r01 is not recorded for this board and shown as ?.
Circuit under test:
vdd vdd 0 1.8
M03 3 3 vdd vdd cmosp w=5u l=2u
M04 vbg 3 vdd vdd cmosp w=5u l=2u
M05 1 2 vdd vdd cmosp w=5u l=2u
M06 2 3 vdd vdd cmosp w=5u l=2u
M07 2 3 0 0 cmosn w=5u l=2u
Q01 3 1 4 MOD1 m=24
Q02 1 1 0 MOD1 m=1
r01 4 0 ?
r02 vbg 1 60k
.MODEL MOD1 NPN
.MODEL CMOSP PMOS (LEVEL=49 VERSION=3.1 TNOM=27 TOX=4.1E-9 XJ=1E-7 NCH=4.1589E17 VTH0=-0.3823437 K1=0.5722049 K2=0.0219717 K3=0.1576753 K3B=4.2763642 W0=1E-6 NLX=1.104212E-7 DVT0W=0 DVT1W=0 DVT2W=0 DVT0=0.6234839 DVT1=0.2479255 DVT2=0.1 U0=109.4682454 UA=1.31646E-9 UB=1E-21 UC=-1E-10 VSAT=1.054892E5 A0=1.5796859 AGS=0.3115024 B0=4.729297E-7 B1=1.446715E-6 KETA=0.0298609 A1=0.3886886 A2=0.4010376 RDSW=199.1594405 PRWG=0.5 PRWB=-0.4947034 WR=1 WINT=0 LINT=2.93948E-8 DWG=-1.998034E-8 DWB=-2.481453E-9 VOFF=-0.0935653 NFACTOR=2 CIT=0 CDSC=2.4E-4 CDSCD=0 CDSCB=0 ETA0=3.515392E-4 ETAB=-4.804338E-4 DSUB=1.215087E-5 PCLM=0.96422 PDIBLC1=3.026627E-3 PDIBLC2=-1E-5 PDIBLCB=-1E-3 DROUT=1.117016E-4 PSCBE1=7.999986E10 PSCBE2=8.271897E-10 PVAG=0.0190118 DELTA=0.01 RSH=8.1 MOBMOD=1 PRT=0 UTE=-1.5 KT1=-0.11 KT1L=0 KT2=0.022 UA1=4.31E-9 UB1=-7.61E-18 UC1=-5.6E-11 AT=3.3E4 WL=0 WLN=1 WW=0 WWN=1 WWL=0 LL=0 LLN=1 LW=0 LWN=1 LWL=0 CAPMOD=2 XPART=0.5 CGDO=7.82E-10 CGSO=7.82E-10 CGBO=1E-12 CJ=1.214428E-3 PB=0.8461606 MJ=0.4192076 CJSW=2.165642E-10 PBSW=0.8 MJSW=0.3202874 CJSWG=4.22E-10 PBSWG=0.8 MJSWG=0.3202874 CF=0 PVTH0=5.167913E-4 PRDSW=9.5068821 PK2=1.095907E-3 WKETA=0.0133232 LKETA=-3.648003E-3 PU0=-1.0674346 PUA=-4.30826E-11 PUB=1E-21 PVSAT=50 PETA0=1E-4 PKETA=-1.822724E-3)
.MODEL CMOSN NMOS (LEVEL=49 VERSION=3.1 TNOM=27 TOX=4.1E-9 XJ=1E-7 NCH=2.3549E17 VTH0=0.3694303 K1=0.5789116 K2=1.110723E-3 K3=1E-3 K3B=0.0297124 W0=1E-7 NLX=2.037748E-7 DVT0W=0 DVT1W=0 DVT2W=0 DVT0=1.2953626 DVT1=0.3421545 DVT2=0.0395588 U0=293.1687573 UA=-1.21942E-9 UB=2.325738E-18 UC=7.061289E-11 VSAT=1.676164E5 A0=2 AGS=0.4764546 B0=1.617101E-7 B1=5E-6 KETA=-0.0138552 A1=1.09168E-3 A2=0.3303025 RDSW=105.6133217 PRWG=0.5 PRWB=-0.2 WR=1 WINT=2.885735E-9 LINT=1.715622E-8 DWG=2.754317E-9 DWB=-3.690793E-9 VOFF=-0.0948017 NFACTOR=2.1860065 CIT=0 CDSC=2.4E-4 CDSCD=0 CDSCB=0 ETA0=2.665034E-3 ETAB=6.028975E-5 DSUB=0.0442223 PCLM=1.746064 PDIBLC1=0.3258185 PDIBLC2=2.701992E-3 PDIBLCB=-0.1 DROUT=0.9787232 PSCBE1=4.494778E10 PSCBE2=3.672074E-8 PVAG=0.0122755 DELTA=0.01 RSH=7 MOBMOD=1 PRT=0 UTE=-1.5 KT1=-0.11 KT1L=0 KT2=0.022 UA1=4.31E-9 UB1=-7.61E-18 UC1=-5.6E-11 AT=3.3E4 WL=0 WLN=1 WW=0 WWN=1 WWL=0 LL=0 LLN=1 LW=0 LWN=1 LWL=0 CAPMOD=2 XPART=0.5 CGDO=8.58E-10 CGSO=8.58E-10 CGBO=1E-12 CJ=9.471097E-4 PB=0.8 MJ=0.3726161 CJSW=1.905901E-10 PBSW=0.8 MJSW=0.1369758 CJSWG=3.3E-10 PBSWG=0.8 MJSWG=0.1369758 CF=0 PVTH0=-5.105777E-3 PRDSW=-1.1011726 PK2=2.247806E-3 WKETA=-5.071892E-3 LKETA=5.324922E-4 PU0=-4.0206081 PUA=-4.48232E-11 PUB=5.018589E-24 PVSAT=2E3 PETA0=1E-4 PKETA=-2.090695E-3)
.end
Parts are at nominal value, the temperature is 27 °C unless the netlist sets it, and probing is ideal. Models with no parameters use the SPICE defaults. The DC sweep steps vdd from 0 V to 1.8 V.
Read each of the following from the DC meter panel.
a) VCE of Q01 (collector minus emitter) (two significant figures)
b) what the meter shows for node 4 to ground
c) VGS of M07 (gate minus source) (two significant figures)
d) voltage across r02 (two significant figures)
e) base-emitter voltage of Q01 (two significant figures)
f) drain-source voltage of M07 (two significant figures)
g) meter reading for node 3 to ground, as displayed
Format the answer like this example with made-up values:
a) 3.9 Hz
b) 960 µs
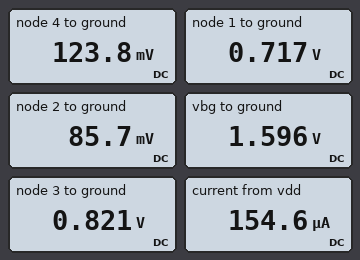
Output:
a) 700 mV
b) 123.8 mV
c) 820 mV
d) 880 mV
e) 590 mV
f) 86 mV
g) 0.821 V
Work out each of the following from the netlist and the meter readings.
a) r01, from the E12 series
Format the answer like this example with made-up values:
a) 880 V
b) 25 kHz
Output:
a) 5.6 kΩ
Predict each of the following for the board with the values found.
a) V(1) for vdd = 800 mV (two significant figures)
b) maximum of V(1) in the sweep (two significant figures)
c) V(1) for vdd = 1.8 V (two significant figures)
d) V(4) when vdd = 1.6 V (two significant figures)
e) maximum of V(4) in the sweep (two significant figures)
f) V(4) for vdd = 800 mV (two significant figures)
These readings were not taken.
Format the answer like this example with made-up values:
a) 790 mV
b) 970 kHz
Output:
a) 610 mV
b) 720 mV
c) 720 mV
d) 110 mV
e) 120 mV
f) 40 mV
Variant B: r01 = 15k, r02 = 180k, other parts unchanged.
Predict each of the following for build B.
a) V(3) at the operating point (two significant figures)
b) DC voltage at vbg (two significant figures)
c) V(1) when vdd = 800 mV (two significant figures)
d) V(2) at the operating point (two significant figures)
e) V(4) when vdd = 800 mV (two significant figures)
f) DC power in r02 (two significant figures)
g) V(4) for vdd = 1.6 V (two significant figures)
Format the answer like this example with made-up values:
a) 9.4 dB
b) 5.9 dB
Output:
a) 1.0 V
b) 1.7 V
c) 590 mV
d) 23 mV
e) 49 mV
f) 5.3 µW
g) 140 mV
